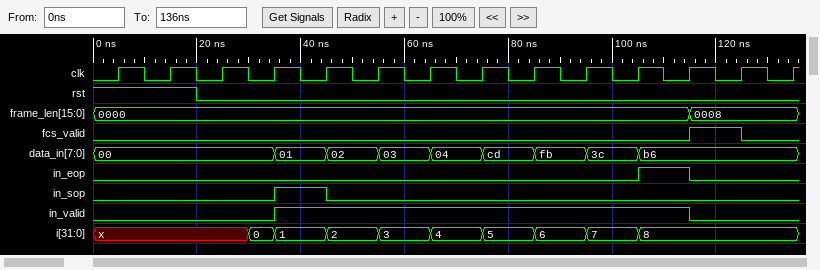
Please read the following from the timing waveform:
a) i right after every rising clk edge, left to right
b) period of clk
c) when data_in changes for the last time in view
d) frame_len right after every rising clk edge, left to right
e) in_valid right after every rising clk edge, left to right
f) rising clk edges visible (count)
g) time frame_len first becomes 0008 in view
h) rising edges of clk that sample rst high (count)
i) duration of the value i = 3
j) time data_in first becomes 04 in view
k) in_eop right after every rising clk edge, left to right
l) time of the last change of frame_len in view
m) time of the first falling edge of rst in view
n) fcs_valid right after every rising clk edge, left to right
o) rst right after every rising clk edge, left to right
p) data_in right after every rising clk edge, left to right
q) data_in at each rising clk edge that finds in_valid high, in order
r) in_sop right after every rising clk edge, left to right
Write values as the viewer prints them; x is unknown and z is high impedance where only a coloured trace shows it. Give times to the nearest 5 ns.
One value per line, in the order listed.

x, x, x, 1, 2, 3, 4, 5, 6, 7, 8, 8, 8, 8
10 ns
105 ns
0000, 0000, 0000, 0000, 0000, 0000, 0000, 0000, 0000, 0000, 0000, 0008, 0008, 0008
0 0 0 1 1 1 1 1 1 1 1 0 0 0
14
115 ns
2
10 ns
65 ns
0 0 0 0 0 0 0 0 0 0 1 0 0 0
115 ns
20 ns
0 0 0 0 0 0 0 0 0 0 0 1 0 0
1 1 0 0 0 0 0 0 0 0 0 0 0 0
00, 00, 00, 01, 02, 03, 04, cd, fb, 3c, b6, b6, b6, b6
01, 02, 03, 04, cd, fb, 3c, b6
0 0 0 1 0 0 0 0 0 0 0 0 0 0
